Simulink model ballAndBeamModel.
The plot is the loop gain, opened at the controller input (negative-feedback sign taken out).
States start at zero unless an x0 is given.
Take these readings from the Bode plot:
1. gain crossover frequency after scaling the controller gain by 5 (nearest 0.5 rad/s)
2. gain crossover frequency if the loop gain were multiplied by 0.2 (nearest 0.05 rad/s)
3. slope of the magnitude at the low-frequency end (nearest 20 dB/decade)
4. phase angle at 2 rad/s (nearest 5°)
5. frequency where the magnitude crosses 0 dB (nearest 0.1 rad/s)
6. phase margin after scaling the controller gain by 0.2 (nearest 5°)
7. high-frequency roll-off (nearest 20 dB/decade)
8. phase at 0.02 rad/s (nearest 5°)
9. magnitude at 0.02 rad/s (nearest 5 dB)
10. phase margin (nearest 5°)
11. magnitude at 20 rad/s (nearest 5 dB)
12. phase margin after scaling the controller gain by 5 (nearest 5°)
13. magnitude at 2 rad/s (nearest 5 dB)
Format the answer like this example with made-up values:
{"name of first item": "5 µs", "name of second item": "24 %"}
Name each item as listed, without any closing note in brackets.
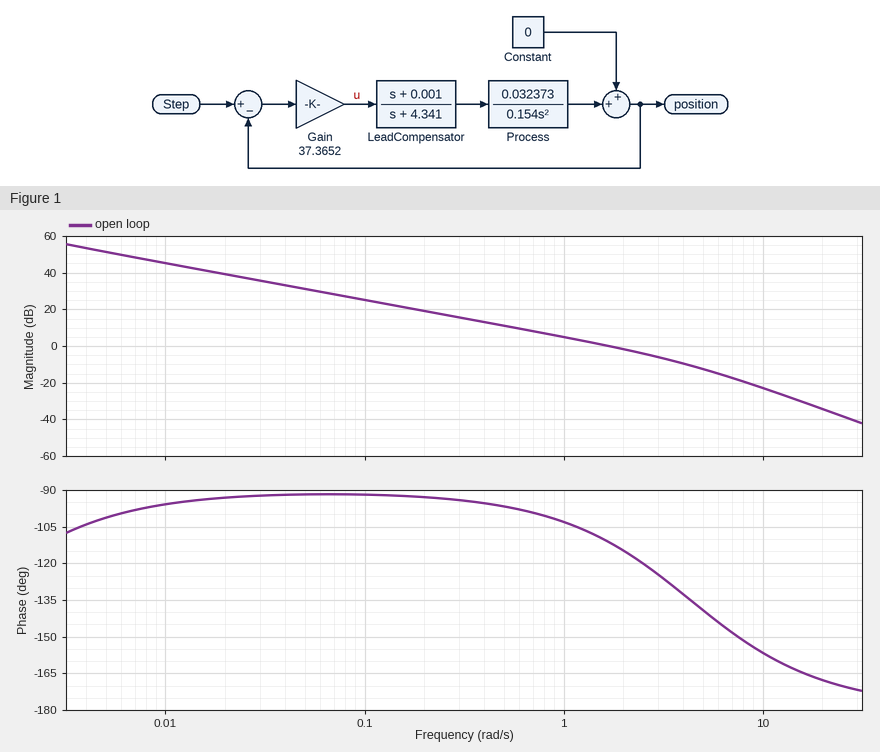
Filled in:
{"gain crossover frequency after scaling the controller gain by 5": "5.5 rad/s", "gain crossover frequency if the loop gain were multiplied by 0.2": "0.35 rad/s", "slope of the magnitude at the low-frequency end": "-20 dB/decade", "phase angle at 2 rad/s": "-115°", "frequency where the magnitude crosses 0 dB": "1.7 rad/s", "phase margin after scaling the controller gain by 0.2": "85°", "high-frequency roll-off": "-40 dB/decade", "phase at 0.02 rad/s": "-95°", "magnitude at 0.02 rad/s": "40 dB", "phase margin": "70°", "magnitude at 20 rad/s": "-35 dB", "phase margin after scaling the controller gain by 5": "40°", "magnitude at 2 rad/s": "0 dB"}
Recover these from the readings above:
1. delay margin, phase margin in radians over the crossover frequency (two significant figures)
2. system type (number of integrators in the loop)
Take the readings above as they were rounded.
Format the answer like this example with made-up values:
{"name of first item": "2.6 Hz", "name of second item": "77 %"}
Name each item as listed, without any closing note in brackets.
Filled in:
{"delay margin, phase margin in radians over the crossover frequency": "0.72 s", "system type": "1"}
